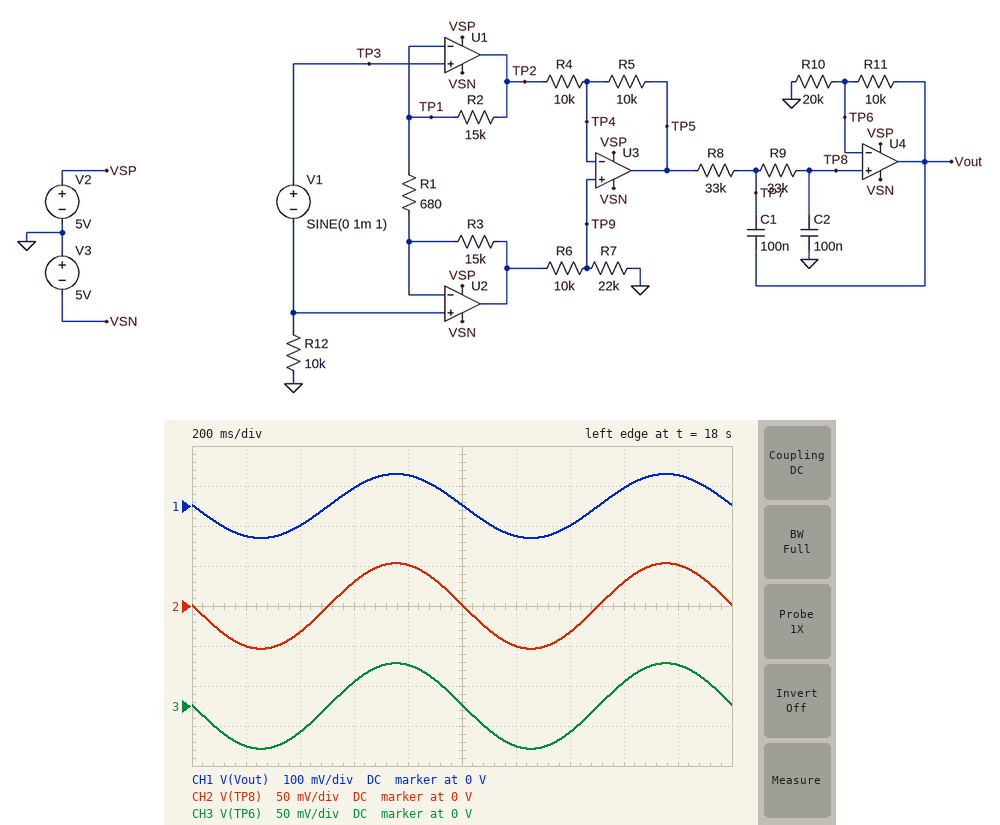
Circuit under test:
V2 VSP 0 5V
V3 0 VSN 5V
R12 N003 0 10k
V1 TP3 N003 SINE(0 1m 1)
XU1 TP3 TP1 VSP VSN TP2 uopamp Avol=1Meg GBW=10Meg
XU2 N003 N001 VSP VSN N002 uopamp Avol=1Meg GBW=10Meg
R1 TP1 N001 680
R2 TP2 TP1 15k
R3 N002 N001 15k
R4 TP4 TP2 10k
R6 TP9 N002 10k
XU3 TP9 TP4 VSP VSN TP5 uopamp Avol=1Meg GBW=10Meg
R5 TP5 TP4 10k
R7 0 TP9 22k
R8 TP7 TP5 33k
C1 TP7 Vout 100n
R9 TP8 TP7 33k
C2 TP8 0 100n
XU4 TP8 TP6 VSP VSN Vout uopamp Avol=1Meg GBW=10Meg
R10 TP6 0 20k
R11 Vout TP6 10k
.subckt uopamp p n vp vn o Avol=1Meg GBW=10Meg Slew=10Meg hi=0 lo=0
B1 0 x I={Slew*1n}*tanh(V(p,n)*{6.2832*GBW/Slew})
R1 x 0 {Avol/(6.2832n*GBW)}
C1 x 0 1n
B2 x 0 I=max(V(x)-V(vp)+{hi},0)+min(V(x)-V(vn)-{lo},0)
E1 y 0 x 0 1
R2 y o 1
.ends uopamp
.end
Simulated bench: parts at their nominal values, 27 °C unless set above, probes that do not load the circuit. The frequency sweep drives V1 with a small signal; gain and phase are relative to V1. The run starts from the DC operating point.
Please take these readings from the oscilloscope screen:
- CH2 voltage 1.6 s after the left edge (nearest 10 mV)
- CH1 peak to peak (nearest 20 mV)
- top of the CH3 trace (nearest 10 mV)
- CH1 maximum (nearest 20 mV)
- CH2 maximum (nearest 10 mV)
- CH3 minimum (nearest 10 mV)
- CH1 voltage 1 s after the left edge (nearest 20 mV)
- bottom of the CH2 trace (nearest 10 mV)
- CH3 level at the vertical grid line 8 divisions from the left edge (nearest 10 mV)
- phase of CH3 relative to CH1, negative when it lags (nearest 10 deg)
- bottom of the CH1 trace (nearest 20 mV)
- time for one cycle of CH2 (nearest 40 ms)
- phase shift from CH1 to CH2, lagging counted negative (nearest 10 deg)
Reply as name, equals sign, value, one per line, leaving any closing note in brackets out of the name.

CH2 voltage 1.6 s after the left edge = 30 mV
CH1 peak to peak = 160 mV
top of the CH3 trace = 50 mV
CH1 maximum = 80 mV
CH2 maximum = 50 mV
CH3 minimum = -50 mV
CH1 voltage 1 s after the left edge = 0 V
bottom of the CH2 trace = -50 mV
CH3 level at the vertical grid line 8 divisions from the left edge = 30 mV
phase of CH3 relative to CH1, negative when it lags = 0 deg
bottom of the CH1 trace = -80 mV
time for one cycle of CH2 = 1.00 s
phase shift from CH1 to CH2, lagging counted negative = 0 deg
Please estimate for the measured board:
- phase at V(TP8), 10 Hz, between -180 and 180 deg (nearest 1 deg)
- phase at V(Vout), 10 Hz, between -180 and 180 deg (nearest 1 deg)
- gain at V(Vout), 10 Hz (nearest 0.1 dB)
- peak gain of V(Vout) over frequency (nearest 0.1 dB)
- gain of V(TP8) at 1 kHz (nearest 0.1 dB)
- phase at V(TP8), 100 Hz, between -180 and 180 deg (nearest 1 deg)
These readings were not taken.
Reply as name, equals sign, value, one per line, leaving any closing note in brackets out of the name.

phase at V(TP8), 10 Hz, between -180 and 180 deg = 162 deg
phase at V(Vout), 10 Hz, between -180 and 180 deg = 162 deg
gain at V(Vout), 10 Hz = 38.0 dB
peak gain of V(Vout) over frequency = 38.1 dB
gain of V(TP8) at 1 kHz = -18.1 dB
phase at V(TP8), 100 Hz, between -180 and 180 deg = 43 deg
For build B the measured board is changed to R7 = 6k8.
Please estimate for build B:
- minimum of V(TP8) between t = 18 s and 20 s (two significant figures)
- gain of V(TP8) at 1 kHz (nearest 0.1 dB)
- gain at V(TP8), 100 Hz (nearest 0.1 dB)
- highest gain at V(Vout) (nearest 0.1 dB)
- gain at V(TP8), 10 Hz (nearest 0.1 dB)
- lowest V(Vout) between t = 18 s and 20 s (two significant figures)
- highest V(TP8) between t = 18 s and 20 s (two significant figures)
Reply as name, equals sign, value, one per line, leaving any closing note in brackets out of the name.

minimum of V(TP8) between t = 18 s and 20 s = -41 mV
gain of V(TP8) at 1 kHz = -20.4 dB
gain at V(TP8), 100 Hz = 19.1 dB
highest gain at V(Vout) = 35.8 dB
gain at V(TP8), 10 Hz = 32.2 dB
lowest V(Vout) between t = 18 s and 20 s = -61 mV
highest V(TP8) between t = 18 s and 20 s = 41 mV
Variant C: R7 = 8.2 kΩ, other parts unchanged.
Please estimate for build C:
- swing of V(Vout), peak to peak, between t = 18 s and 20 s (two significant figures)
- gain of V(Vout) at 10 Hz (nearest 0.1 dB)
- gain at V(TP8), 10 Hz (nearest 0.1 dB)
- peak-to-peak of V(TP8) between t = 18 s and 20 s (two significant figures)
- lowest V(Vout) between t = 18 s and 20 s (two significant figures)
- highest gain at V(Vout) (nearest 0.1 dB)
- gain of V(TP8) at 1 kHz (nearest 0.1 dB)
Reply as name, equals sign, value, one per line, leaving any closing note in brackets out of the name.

swing of V(Vout), peak to peak, between t = 18 s and 20 s = 130 mV
gain of V(Vout) at 10 Hz = 36.1 dB
gain at V(TP8), 10 Hz = 32.6 dB
peak-to-peak of V(TP8) between t = 18 s and 20 s = 86 mV
lowest V(Vout) between t = 18 s and 20 s = -64 mV
highest gain at V(Vout) = 36.2 dB
gain of V(TP8) at 1 kHz = -20.0 dB
